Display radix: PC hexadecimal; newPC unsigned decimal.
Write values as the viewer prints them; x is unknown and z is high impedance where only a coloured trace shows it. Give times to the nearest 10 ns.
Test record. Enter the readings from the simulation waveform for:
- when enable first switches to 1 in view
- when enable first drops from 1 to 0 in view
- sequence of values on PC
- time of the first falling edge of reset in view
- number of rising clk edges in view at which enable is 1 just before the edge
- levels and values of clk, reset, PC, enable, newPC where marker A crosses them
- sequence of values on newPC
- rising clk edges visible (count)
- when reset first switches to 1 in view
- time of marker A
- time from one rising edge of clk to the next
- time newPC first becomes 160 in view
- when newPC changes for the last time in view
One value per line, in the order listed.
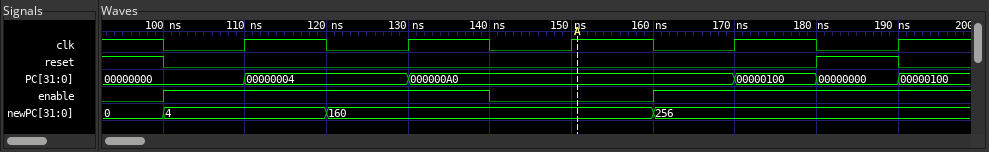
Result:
100 ns
140 ns
00000000, 00000004, 000000A0, 00000100, 00000000, 00000100
100 ns
4
clk=1, reset=0, PC=000000A0, enable=0, newPC=160
0, 4, 160, 256
5
180 ns
150 ns
20 ns
120 ns
160 ns
